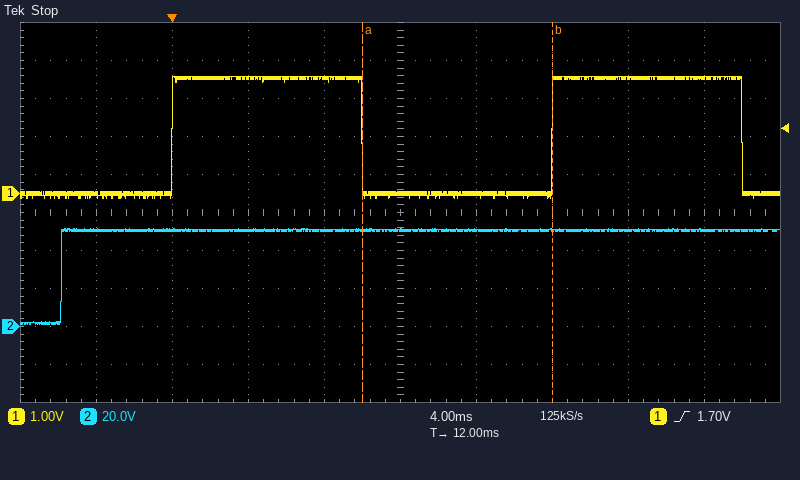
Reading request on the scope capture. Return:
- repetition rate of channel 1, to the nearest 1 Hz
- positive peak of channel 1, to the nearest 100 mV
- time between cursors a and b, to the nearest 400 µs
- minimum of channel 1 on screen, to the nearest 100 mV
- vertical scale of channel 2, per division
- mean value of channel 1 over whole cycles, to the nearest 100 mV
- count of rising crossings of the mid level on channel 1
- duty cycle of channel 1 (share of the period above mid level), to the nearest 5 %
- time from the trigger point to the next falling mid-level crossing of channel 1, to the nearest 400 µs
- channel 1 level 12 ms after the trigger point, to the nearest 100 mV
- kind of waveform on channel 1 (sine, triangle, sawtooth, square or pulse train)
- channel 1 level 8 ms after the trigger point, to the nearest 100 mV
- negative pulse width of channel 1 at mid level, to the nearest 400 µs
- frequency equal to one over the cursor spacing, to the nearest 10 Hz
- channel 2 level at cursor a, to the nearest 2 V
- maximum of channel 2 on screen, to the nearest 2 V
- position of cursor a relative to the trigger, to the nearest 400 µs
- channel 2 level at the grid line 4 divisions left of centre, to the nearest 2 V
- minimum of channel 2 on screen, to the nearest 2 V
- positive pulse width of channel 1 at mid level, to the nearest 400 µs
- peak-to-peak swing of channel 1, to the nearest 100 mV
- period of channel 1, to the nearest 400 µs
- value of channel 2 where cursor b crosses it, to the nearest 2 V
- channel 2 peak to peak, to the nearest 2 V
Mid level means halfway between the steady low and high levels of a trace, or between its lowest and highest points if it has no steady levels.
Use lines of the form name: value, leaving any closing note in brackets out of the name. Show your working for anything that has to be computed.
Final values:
repetition rate of channel 1, to the nearest 1 Hz: 1 / 20.0 ms ≈ 50 Hz
positive peak of channel 1, to the nearest 100 mV: 3.1 V
time between cursors a and b, to the nearest 400 µs: 10.0 ms
minimum of channel 1 on screen, to the nearest 100 mV: -100 mV
vertical scale of channel 2, per division: 20 V
mean value of channel 1 over whole cycles, to the nearest 100 mV: -100 mV + 0.5 × (3.1 V − (-100 mV)) ≈ 1.5 V
count of rising crossings of the mid level on channel 1: 2
duty cycle of channel 1 (share of the period above mid level), to the nearest 5 %: 10.0 ms / 20.0 ms ≈ 50 %
time from the trigger point to the next falling mid-level crossing of channel 1, to the nearest 400 µs: 10.0 ms
channel 1 level 12 ms after the trigger point, to the nearest 100 mV: 0.0 V
kind of waveform on channel 1: square
channel 1 level 8 ms after the trigger point, to the nearest 100 mV: 3.0 V
negative pulse width of channel 1 at mid level, to the nearest 400 µs: 10.0 ms
frequency equal to one over the cursor spacing, to the nearest 10 Hz: 1 / 10.0 ms ≈ 100 Hz
channel 2 level at cursor a, to the nearest 2 V: 50 V
maximum of channel 2 on screen, to the nearest 2 V: 52 V
position of cursor a relative to the trigger, to the nearest 400 µs: +10.0 ms
channel 2 level at the grid line 4 divisions left of centre, to the nearest 2 V: 50 V
minimum of channel 2 on screen, to the nearest 2 V: 2 V
positive pulse width of channel 1 at mid level, to the nearest 400 µs: 10.0 ms
peak-to-peak swing of channel 1, to the nearest 100 mV: 3.1 V − (-100 mV) = 3.2 V
period of channel 1, to the nearest 400 µs: 20.0 ms
value of channel 2 where cursor b crosses it, to the nearest 2 V: 50 V
channel 2 peak to peak, to the nearest 2 V: 52 V − (2 V) = 50 V
